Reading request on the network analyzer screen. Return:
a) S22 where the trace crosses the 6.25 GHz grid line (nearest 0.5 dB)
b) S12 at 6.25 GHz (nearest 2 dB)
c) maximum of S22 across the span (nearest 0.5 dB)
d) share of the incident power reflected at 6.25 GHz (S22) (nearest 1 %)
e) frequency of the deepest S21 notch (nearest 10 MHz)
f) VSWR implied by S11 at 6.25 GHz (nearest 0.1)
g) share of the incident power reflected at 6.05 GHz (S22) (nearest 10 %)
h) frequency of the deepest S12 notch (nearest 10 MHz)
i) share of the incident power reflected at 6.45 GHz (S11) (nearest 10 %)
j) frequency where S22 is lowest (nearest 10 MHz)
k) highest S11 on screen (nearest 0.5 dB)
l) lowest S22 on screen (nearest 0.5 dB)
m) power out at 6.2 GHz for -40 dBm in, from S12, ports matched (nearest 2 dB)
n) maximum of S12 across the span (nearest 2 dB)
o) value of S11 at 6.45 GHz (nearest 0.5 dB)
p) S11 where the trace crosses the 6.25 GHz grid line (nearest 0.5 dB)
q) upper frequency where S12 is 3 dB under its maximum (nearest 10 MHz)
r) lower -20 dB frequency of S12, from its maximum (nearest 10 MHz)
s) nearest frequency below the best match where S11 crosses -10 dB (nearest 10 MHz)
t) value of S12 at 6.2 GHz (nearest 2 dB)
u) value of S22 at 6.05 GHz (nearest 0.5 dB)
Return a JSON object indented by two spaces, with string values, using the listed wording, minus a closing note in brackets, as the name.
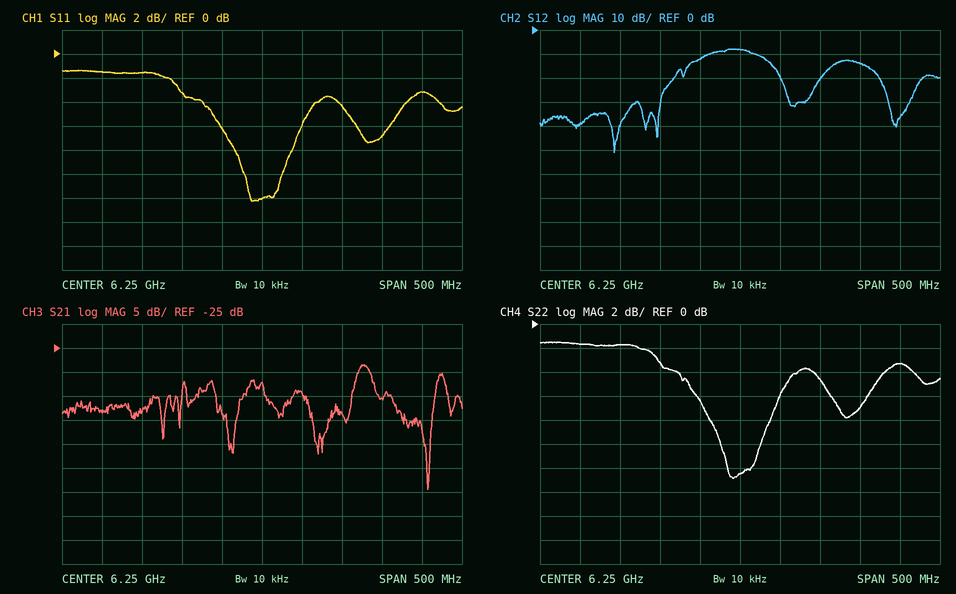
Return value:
{
  "S22 where the trace crosses the 6.25 GHz grid line": "-12.5 dB",
  "S12 at 6.25 GHz": "-8 dB",
  "maximum of S22 across the span": "-1.5 dB",
  "share of the incident power reflected at 6.25 GHz (S22)": "6 %",
  "frequency of the deepest S21 notch": "6.46 GHz",
  "VSWR implied by S11 at 6.25 GHz": "1.7",
  "share of the incident power reflected at 6.05 GHz (S22)": "70 %",
  "frequency of the deepest S12 notch": "6.09 GHz",
  "share of the incident power reflected at 6.45 GHz (S11)": "50 %",
  "frequency where S22 is lowest": "6.24 GHz",
  "highest S11 on screen": "-1.5 dB",
  "lowest S22 on screen": "-13.0 dB",
  "power out at 6.2 GHz for -40 dBm in, from S12, ports matched": "-52 dBm",
  "maximum of S12 across the span": "-8 dB",
  "value of S11 at 6.45 GHz": "-3.0 dB",
  "S11 where the trace crosses the 6.25 GHz grid line": "-12.0 dB",
  "upper frequency where S12 is 3 dB under its maximum": "6.28 GHz",
  "lower -20 dB frequency of S12, from its maximum": "6.15 GHz",
  "nearest frequency below the best match where S11 crosses -10 dB": "6.23 GHz",
  "value of S12 at 6.2 GHz": "-12 dB",
  "value of S22 at 6.05 GHz": "-1.5 dB"
}
